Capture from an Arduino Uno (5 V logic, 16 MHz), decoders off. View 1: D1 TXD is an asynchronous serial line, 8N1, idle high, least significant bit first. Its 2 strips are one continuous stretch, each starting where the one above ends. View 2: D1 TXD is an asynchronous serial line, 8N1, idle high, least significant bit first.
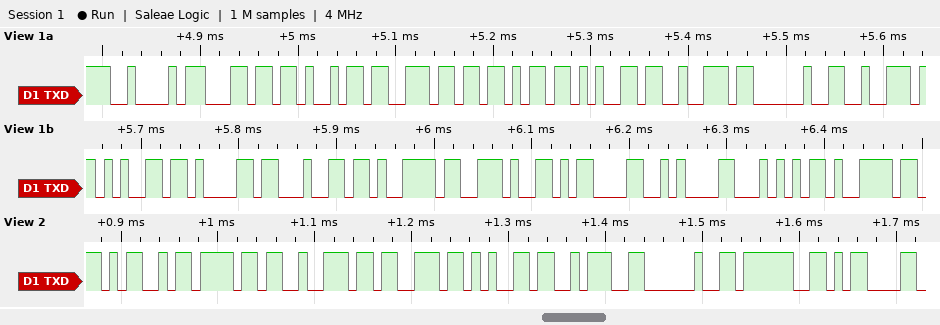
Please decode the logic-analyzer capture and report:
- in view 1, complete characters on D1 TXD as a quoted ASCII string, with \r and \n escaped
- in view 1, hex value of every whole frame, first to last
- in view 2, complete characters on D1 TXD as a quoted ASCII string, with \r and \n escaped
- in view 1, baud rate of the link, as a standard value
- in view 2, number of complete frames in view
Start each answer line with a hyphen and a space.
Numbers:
- "Blinker ready.\r\nTy"
- 42 6C 69 6E 6B 65 72 20 72 65 61 64 79 2E 0D 0A 54 79
- "Morse: ?\r"
- 115200 baud
- 9
